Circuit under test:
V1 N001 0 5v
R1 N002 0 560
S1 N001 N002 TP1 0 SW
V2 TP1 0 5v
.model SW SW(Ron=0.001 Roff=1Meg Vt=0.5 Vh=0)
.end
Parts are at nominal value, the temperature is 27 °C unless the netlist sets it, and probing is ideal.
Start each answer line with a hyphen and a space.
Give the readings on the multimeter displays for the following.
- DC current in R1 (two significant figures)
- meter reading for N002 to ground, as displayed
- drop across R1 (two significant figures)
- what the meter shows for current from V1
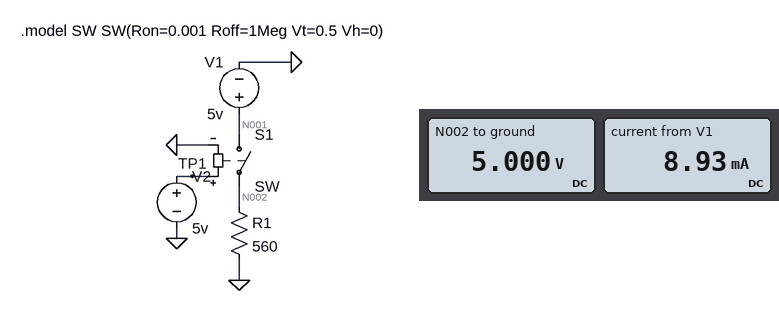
- 8.9 mA
- 5.000 V
- 5.0 V
- 8.93 mA
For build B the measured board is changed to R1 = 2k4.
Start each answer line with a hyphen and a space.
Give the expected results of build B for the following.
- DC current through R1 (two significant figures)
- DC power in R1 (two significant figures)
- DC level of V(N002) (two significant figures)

- 2.1 mA
- 10 mW
- 5.0 V
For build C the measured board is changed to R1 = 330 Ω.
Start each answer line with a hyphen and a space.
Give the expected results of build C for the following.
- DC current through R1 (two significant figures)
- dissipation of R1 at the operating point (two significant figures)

- 15 mA
- 76 mW
